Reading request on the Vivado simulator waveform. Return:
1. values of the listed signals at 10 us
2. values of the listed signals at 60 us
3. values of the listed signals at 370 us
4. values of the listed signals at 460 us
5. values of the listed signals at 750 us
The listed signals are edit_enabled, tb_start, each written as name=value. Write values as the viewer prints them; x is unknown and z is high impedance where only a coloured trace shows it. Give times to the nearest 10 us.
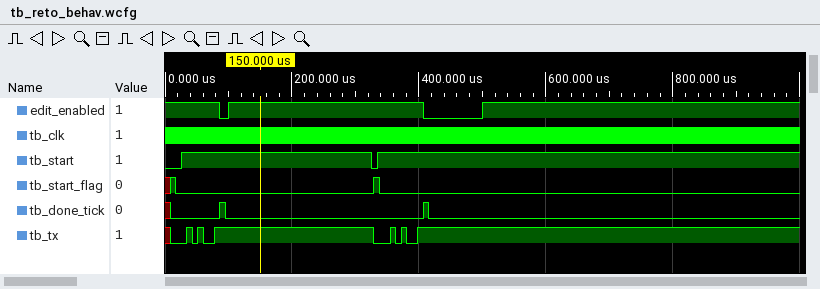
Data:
edit_enabled=1, tb_start=0
edit_enabled=1, tb_start=1
edit_enabled=1, tb_start=1
edit_enabled=0, tb_start=1
edit_enabled=1, tb_start=1
